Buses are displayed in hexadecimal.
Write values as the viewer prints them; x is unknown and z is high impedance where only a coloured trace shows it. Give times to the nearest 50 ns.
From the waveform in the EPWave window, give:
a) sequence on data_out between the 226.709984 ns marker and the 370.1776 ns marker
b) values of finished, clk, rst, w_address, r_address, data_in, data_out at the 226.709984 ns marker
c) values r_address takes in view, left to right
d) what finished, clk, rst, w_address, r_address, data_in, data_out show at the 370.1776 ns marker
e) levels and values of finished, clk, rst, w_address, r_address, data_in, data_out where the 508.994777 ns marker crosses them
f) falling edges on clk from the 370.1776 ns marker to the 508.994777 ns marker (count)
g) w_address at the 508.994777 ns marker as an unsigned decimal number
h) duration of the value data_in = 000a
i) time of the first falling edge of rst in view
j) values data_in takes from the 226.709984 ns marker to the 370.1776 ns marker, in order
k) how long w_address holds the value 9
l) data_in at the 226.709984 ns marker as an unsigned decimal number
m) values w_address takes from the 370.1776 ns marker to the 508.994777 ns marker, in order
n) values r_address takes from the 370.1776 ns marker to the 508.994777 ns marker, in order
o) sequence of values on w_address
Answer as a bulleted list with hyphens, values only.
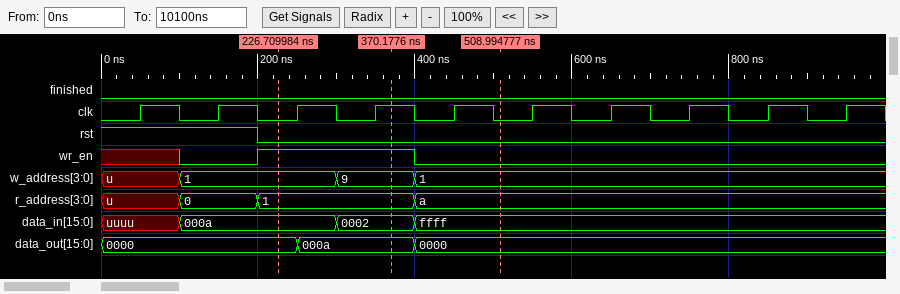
- 0000, 000a
- finished=0, clk=0, rst=0, w_address=1, r_address=1, data_in=000a, data_out=0000
- u, 0, 1, a
- finished=0, clk=1, rst=0, w_address=9, r_address=1, data_in=0002, data_out=000a
- finished=0, clk=0, rst=0, w_address=1, r_address=a, data_in=ffff, data_out=0000
- 2
- 1
- 200 ns
- 200 ns
- 000a, 0002
- 100 ns
- 10
- 9, 1
- 1, a
- u, 1, 9, 1
